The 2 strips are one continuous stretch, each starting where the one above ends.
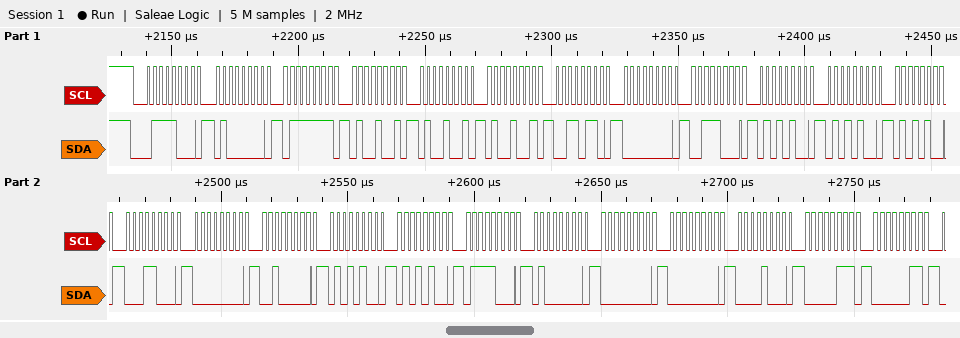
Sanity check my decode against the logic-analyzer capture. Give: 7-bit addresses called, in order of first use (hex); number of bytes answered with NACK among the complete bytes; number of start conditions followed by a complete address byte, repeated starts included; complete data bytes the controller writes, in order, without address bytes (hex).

0x3C
0
1
40 7F 49 49 49 36 00 38 54 54 54 18 00 20 54 54 78 40 00 00 08 07 03
